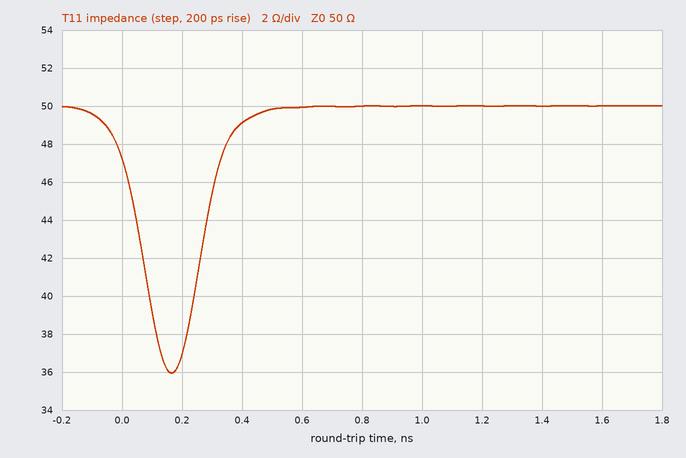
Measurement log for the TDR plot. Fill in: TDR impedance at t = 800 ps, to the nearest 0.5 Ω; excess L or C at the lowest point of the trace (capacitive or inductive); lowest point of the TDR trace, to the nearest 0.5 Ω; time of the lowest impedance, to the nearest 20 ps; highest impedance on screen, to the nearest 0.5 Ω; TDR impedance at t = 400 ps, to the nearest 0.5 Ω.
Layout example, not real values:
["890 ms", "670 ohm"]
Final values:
["50.0 Ω", "capacitive", "36.0 Ω", "160 ps", "50.0 Ω", "49.0 Ω"]
